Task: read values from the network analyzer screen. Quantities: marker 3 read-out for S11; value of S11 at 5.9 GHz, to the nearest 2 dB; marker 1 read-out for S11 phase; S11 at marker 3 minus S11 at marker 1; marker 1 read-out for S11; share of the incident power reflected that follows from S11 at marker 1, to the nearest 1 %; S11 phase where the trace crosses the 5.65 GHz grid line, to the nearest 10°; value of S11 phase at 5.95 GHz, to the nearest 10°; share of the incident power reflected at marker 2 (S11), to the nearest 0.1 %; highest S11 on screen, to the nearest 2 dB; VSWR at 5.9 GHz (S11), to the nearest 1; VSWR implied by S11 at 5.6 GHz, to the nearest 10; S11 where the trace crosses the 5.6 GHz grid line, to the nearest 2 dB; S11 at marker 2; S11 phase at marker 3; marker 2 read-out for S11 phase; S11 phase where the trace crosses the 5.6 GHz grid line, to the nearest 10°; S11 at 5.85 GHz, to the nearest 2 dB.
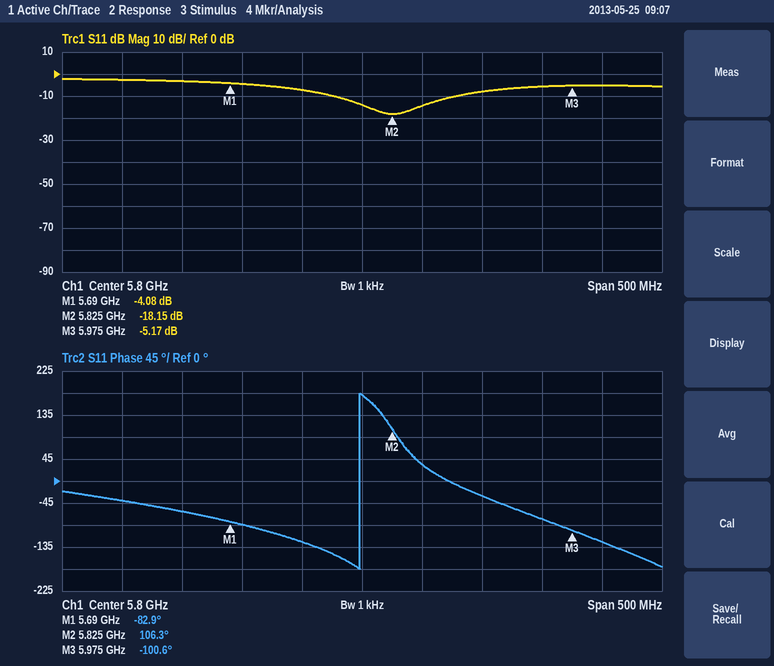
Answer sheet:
-5.17 dB
-8 dB
-82.9°
-1.09 dB
-4.08 dB
39 %
-60°
-80°
1.5 %
-2 dB
2
10
-2 dB
-18.15 dB
-100.6°
106.3°
-40°
-14 dB
